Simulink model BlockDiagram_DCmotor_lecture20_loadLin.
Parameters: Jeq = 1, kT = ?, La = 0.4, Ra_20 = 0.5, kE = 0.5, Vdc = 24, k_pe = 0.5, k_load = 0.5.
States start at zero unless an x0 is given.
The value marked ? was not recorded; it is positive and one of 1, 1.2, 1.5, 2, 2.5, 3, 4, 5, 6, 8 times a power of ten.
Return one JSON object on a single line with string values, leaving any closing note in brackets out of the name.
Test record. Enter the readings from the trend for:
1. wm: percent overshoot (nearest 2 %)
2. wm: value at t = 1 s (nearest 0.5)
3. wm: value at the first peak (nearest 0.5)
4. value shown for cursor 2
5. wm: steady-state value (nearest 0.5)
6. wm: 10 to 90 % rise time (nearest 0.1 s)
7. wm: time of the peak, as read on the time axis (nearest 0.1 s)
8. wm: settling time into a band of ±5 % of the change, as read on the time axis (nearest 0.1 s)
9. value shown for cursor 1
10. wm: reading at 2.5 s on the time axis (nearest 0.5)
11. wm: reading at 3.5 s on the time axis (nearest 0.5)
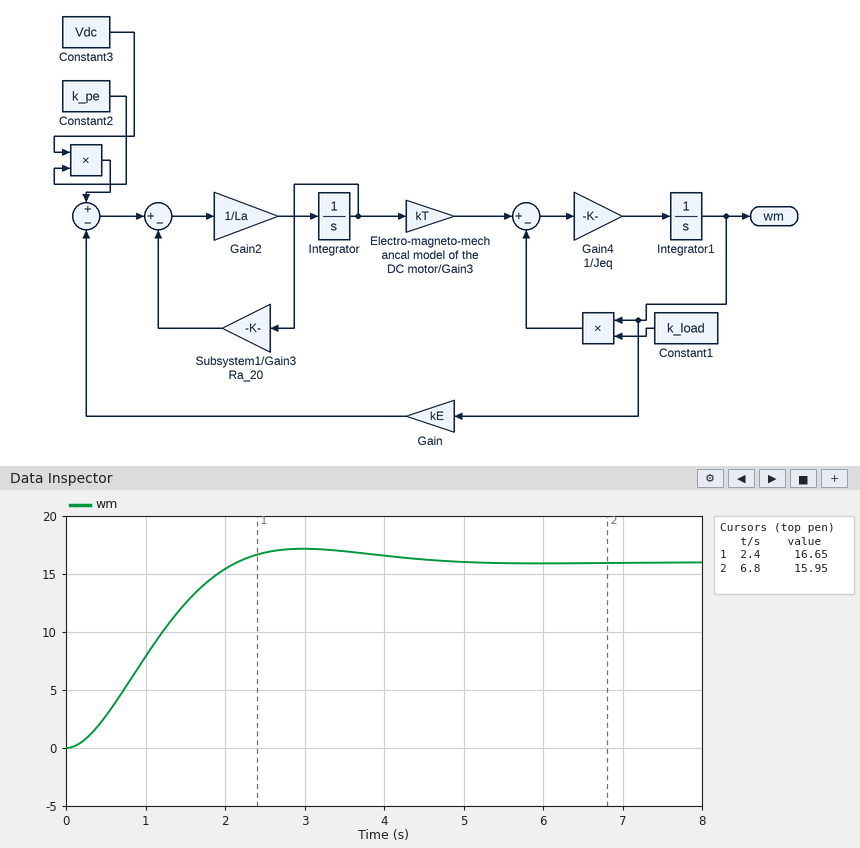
{"wm: percent overshoot": "8 %", "wm: value at t = 1 s": "8.0", "wm: value at the first peak": "17.0", "value shown for cursor 2": "15.95", "wm: steady-state value": "16.0", "wm: 10 to 90 % rise time": "1.4 s", "wm: time of the peak, as read on the time axis": "3.0 s", "wm: settling time into a band of ±5 % of the change, as read on the time axis": "3.7 s", "value shown for cursor 1": "16.65", "wm: reading at 2.5 s on the time axis": "17.0", "wm: reading at 3.5 s on the time axis": "17.0"}
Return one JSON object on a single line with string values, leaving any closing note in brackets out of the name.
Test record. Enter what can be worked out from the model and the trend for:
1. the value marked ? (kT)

{"the value marked ?": "1"}
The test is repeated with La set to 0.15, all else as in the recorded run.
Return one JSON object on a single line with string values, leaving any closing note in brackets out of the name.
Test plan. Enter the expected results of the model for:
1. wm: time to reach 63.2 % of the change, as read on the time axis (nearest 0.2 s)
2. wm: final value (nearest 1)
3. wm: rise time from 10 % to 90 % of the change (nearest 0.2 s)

{"wm: time to reach 63.2 % of the change, as read on the time axis": "0.8 s", "wm: final value": "16", "wm: rise time from 10 % to 90 % of the change": "1.2 s"}
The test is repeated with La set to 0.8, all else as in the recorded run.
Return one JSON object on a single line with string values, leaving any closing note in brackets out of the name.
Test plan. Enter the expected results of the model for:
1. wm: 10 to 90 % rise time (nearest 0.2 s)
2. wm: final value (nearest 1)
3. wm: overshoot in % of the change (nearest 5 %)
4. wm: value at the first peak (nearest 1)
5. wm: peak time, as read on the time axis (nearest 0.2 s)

{"wm: 10 to 90 % rise time": "1.8 s", "wm: final value": "16", "wm: overshoot in % of the change": "10 %", "wm: value at the first peak": "18", "wm: peak time, as read on the time axis": "4.0 s"}
